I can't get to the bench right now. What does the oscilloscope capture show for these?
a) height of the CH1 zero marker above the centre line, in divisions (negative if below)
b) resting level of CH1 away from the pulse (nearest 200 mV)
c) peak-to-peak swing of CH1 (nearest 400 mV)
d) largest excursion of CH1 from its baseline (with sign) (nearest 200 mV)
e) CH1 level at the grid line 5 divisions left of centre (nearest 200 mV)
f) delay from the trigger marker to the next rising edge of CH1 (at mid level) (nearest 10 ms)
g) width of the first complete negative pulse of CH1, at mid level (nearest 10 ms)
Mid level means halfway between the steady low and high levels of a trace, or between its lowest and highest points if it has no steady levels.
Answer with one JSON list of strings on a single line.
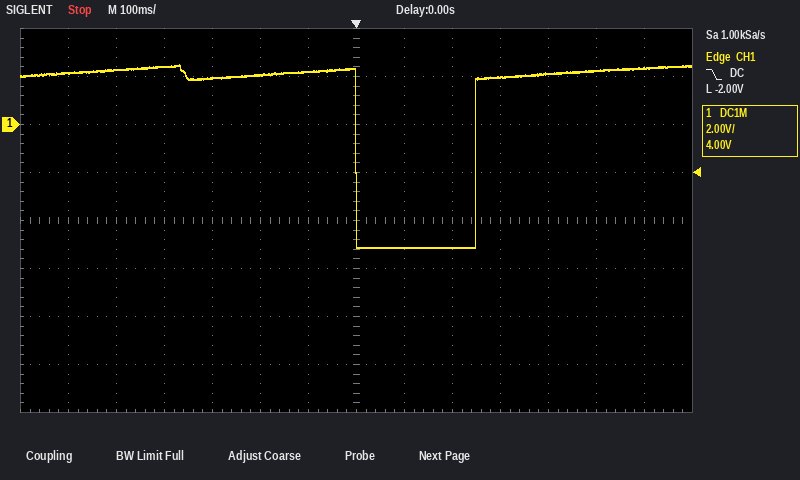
["+2.0 div", "2.2 V", "7.6 V", "-7.2 V", "2.2 V", "250 ms", "250 ms"]
